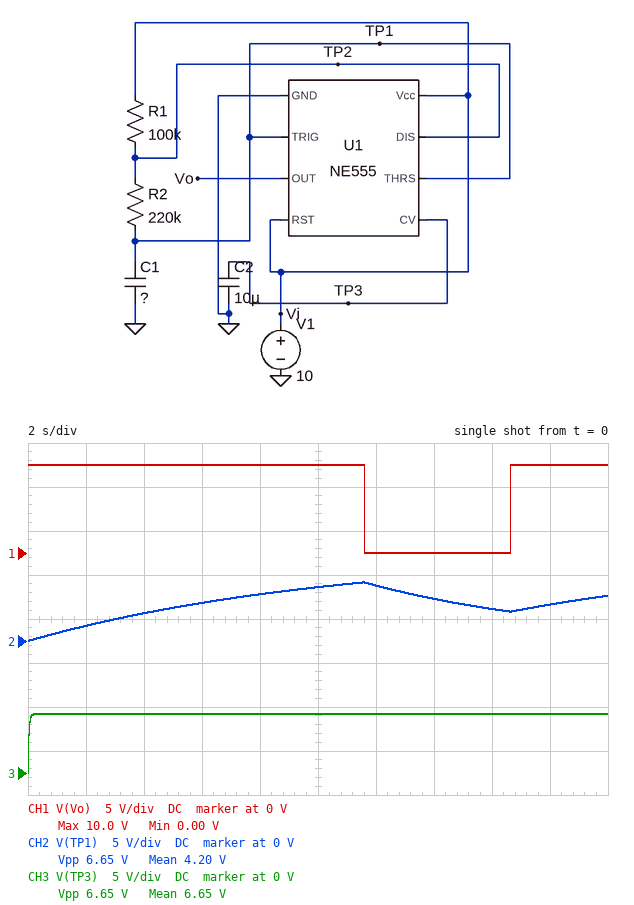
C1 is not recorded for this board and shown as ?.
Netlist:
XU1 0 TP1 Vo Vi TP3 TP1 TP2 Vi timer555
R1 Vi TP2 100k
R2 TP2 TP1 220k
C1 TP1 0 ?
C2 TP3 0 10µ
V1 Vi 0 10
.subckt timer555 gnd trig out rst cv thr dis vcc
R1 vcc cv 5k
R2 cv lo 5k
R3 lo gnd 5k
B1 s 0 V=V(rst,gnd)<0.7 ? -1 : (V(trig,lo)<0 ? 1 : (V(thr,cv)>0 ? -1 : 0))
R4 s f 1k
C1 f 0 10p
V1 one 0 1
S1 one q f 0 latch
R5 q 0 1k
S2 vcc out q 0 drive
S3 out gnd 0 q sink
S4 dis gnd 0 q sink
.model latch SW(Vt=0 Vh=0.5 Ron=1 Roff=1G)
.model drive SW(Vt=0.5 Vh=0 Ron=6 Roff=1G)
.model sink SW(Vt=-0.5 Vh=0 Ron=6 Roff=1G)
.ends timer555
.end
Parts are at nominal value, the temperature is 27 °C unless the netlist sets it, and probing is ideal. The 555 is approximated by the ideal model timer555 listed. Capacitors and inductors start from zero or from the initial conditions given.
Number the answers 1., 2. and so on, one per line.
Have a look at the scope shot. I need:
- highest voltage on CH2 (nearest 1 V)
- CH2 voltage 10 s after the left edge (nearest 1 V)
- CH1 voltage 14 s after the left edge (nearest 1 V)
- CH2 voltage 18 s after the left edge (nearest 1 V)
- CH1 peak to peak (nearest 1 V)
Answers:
1. 7 V
2. 6 V
3. 0 V
4. 4 V
5. 10 V
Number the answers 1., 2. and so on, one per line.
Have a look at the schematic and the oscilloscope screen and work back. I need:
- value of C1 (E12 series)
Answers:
1. 33 µF
